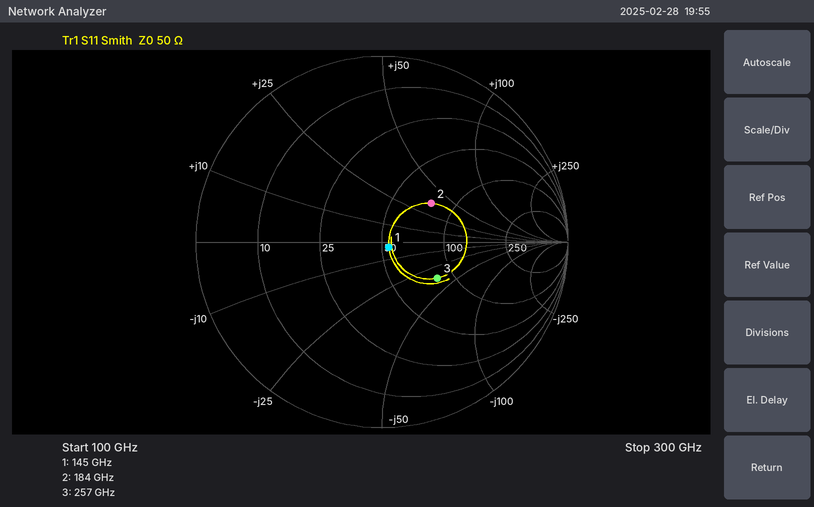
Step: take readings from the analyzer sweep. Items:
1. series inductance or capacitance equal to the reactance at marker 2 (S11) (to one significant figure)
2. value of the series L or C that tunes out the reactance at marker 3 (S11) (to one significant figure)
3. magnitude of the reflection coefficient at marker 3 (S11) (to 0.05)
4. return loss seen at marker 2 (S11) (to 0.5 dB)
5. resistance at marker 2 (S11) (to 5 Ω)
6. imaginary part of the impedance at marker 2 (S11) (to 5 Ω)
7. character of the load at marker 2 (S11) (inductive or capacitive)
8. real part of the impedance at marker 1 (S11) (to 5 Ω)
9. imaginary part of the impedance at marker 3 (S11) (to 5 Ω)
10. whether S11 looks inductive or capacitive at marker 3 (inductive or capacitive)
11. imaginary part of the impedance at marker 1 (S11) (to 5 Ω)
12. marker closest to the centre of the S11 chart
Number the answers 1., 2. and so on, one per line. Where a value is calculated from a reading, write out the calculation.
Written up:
1. L = 35 Ω/(2π × 184 GHz) ≈ 30 pH
2. L = 35 Ω/(2π × 257 GHz) ≈ 21.7 pH, so 20 pH to one significant figure
3. 0.35
4. 9.5 dB
5. 75 Ω
6. +35 Ω
7. inductive
8. 55 Ω
9. -35 Ω
10. capacitive
11. -5 Ω
12. marker 1
